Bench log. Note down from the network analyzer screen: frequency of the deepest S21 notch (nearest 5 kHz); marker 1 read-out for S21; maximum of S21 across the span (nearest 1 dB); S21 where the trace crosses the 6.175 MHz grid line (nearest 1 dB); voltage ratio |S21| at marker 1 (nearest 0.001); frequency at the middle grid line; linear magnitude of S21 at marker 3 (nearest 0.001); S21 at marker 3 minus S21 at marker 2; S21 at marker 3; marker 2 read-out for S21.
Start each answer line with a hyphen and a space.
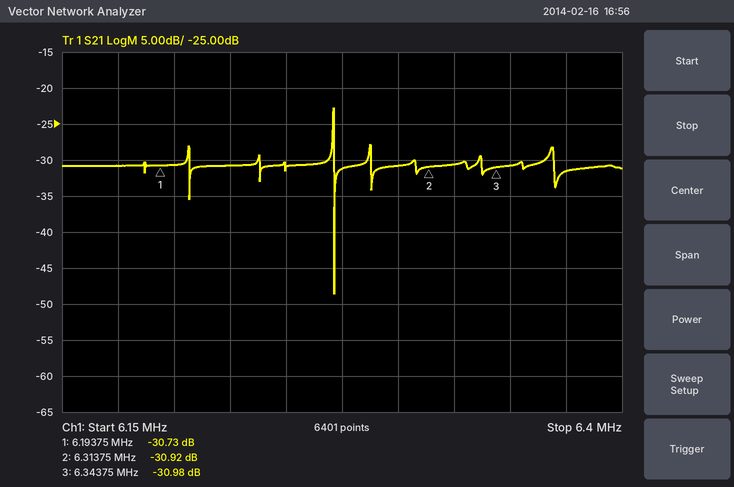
- 6.270 MHz
- -30.73 dB
- -23 dB
- -31 dB
- 0.029
- 6.275 MHz
- 0.028
- -0.06 dB
- -30.98 dB
- -30.92 dB
